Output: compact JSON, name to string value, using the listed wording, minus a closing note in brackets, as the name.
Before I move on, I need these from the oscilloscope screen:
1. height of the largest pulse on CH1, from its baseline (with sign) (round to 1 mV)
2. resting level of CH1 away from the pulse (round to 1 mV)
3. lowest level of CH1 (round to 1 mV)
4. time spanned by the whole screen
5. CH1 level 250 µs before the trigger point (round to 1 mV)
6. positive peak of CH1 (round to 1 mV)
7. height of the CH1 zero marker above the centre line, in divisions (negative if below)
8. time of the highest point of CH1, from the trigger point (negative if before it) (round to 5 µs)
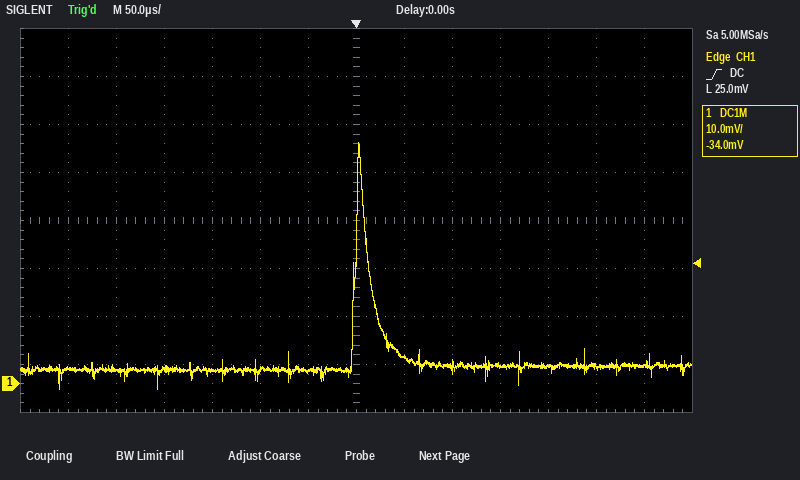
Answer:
{"height of the largest pulse on CH1, from its baseline (with sign)": "+47 mV", "resting level of CH1 away from the pulse": "3 mV", "lowest level of CH1": "-1 mV", "time spanned by the whole screen": "700 µs", "CH1 level 250 µs before the trigger point": "3 mV", "positive peak of CH1": "50 mV", "height of the CH1 zero marker above the centre line, in divisions": "-3.4 div", "time of the highest point of CH1, from the trigger point (negative if before it)": "+5 µs"}
